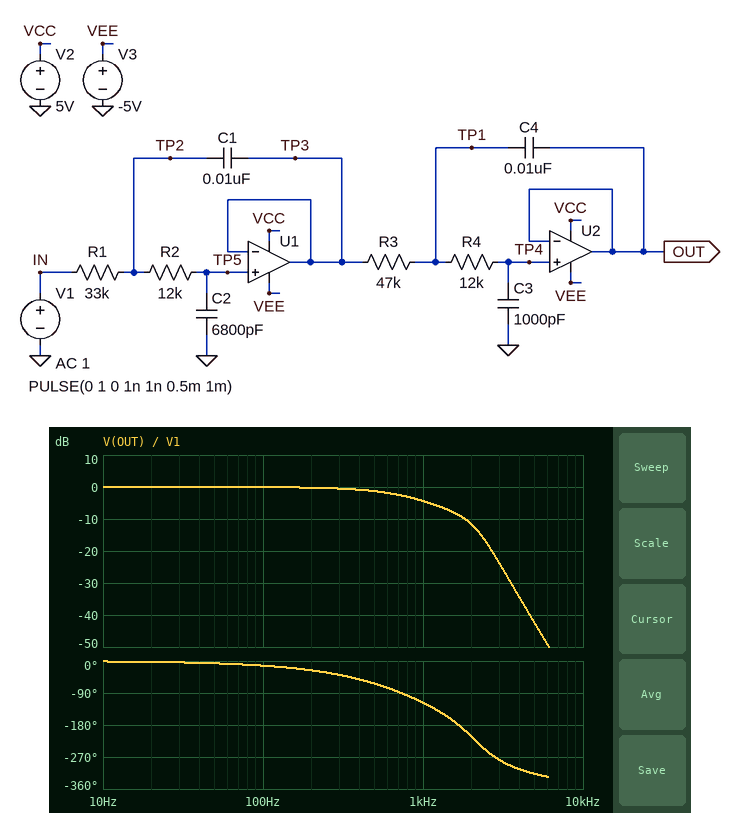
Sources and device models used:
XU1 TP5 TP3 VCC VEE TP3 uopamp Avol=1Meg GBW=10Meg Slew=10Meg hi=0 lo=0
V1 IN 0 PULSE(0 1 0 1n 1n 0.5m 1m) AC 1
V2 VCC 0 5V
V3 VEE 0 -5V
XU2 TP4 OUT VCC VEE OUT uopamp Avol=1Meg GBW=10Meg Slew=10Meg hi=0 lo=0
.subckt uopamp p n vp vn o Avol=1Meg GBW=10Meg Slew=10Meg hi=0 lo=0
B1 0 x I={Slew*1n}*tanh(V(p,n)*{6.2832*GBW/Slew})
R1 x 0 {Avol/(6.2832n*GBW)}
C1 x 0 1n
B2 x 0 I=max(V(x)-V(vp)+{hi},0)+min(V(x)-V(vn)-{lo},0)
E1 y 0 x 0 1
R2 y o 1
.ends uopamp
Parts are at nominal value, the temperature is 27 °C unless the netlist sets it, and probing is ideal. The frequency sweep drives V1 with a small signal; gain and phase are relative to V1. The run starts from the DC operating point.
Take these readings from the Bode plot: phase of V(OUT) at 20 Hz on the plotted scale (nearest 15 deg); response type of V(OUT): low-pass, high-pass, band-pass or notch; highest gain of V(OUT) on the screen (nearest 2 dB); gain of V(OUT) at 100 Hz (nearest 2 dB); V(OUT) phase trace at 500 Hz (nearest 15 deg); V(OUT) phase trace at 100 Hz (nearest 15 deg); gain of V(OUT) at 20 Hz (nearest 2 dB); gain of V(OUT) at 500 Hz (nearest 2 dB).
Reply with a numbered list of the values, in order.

1. 0 deg
2. low-pass
3. 0 dB
4. 0 dB
5. -60 deg
6. -15 deg
7. 0 dB
8. -2 dB
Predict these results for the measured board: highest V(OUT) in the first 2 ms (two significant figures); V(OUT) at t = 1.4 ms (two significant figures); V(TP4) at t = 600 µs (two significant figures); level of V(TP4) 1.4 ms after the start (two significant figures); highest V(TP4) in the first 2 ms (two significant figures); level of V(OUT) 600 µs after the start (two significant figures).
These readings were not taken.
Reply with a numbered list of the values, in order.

1. 880 mV
2. 680 mV
3. 880 mV
4. 680 mV
5. 880 mV
6. 880 mV
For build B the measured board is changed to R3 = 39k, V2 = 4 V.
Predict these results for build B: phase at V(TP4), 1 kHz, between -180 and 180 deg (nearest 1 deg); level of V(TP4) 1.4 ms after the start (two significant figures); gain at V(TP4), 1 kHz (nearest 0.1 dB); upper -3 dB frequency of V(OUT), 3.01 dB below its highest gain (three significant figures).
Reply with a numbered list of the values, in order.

1. -113 deg
2. 700 mV
3. -4.5 dB
4. 774 Hz
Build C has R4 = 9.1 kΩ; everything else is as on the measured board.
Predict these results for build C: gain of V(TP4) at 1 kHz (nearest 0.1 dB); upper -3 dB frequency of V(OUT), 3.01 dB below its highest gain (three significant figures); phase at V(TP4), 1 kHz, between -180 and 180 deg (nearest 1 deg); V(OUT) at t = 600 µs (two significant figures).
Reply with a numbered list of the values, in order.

1. -4.8 dB
2. 753 Hz
3. -115 deg
4. 870 mV
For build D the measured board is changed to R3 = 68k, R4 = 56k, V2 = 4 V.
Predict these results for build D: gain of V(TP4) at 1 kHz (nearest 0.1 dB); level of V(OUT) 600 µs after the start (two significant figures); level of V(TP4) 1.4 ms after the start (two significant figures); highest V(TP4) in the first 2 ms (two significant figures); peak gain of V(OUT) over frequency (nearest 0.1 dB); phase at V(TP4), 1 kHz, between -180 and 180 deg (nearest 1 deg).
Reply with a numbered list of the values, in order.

1. -5.0 dB
2. 730 mV
3. 110 mV
4. 960 mV
5. 1.4 dB
6. 145 deg
